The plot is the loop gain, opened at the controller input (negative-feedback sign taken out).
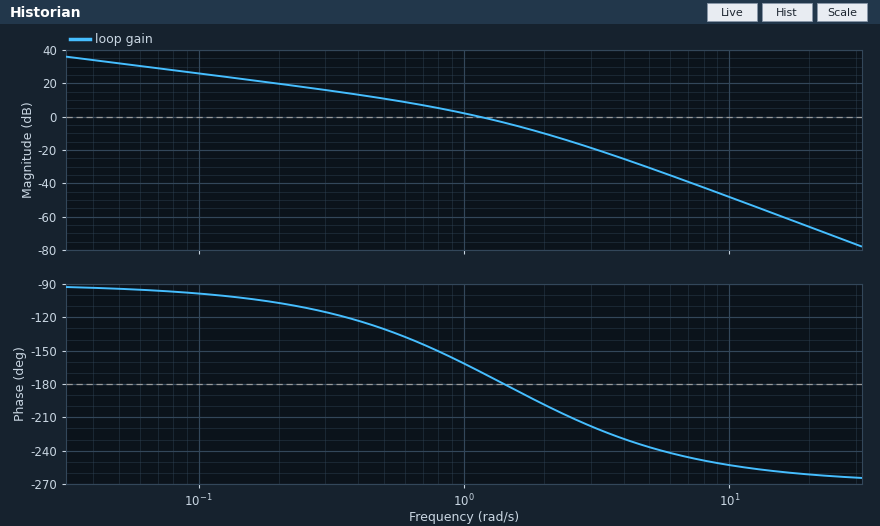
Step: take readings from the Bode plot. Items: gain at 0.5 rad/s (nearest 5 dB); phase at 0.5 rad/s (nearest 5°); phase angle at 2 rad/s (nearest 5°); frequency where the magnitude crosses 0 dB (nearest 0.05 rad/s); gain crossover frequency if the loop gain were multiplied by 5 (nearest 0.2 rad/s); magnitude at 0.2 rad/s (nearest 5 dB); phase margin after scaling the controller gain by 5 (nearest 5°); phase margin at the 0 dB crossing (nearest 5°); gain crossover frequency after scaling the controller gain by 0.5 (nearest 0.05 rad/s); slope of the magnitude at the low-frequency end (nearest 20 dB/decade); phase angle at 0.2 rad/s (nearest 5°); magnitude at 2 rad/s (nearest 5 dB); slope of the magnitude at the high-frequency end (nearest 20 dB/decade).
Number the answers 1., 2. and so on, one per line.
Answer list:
1. 10 dB
2. -130°
3. -200°
4. 1.15 rad/s
5. 2.4 rad/s
6. 20 dB
7. -30°
8. 10°
9. 0.75 rad/s
10. -20 dB/decade
11. -105°
12. -10 dB
13. -60 dB/decade
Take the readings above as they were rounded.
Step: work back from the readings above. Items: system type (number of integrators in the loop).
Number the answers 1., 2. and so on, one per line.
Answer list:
1. 1
